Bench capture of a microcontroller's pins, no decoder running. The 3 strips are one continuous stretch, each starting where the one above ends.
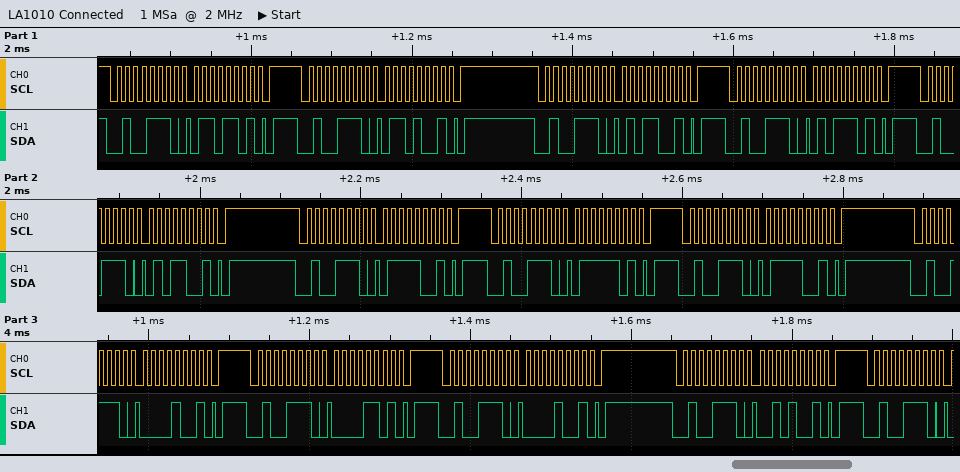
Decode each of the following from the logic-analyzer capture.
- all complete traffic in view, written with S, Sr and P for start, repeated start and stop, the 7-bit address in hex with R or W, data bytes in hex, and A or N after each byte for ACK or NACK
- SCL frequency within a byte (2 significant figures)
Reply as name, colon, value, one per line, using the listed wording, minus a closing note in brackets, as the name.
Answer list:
all complete traffic in view, written with S, Sr and P for start, repeated start and stop, the 7-bit address in hex with R or W, data bytes in hex, and A or N after each byte for ACK or NACK: S 27W A 6D A P S 27W A 69 A P S 27W A 59 A P S 27W A 5D A P S 27W A 59 A P S 27W A 79 A P S 27W A 7D A P S 27W A 79 A P S 27W A 09 A P S 27W A 0D A P S 27W A 09 A P S 27W A 29 A P S 27W A
SCL frequency within a byte: 100 kHz
